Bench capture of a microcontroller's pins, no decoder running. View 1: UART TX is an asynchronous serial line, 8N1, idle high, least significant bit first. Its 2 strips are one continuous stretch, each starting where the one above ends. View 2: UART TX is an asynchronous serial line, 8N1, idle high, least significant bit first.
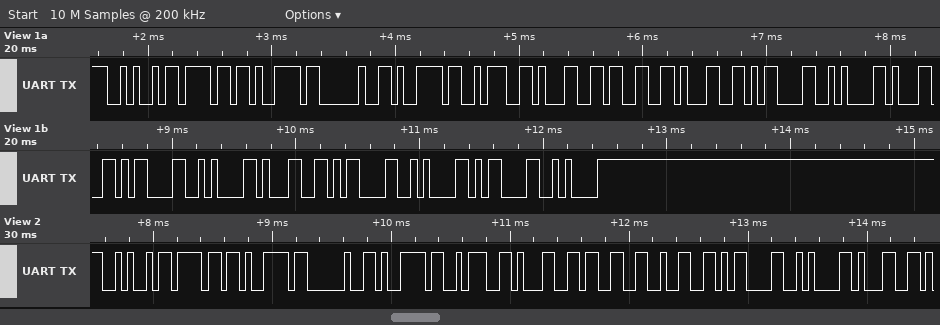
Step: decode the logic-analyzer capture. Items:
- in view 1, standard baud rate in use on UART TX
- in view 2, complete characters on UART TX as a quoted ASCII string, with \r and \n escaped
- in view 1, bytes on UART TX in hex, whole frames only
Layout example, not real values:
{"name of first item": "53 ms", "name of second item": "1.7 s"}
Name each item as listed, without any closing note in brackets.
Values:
{"in view 1, standard baud rate in use on UART TX": "19200 baud", "in view 2, complete characters on UART TX as a quoted ASCII string, with \\r and \\n escaped": "\"Joy y:132\\r\\n1\"", "in view 1, bytes on UART TX in hex, whole frames only": "4A 6F 79 20 79 3A 31 33 31 0D 0A 31 0D 0A 31 0D 0A 0D 0A"}
